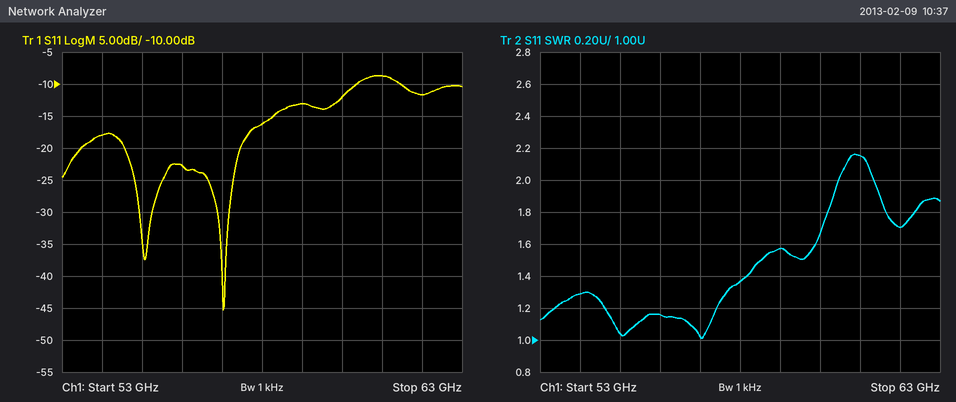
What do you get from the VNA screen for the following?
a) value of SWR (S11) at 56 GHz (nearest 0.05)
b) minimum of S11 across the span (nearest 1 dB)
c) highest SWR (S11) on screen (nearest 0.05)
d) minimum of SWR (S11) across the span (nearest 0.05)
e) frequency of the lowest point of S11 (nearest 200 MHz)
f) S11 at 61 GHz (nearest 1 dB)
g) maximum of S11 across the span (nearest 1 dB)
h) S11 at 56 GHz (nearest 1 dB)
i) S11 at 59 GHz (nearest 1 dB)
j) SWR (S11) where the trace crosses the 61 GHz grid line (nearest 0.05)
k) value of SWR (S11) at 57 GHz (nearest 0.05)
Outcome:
1.15
-45 dB
2.15
1.00
57.0 GHz
-9 dB
-9 dB
-23 dB
-13 dB
2.15
1.00
